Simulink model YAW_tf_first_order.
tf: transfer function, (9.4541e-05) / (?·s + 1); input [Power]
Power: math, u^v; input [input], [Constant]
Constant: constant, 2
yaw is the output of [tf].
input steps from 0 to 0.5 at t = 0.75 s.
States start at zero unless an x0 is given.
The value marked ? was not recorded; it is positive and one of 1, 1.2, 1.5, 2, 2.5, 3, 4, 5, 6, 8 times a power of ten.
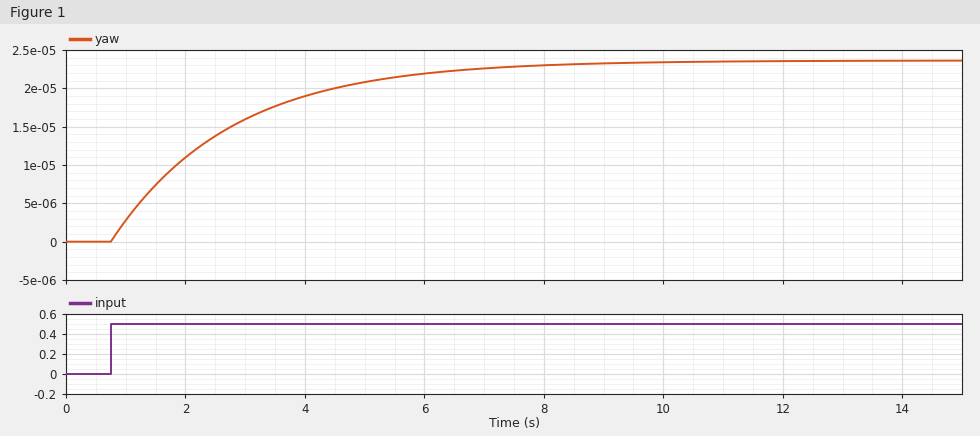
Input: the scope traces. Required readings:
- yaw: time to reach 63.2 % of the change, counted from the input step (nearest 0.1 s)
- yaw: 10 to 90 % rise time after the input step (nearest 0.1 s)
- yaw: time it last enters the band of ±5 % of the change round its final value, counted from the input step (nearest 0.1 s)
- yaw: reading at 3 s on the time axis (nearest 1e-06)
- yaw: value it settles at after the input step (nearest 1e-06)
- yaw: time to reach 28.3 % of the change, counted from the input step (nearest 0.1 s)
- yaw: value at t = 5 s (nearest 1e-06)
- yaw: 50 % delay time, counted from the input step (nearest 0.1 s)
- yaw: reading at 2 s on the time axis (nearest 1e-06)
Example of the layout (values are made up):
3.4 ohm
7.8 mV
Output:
2.0 s
4.4 s
6.0 s
0.000016
0.000024
0.7 s
0.000021
1.4 s
0.000011
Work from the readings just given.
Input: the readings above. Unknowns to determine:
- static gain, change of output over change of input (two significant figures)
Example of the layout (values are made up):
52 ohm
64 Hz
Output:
0.000048
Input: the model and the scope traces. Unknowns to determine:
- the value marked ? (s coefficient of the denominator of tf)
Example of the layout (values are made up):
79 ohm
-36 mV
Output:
2
